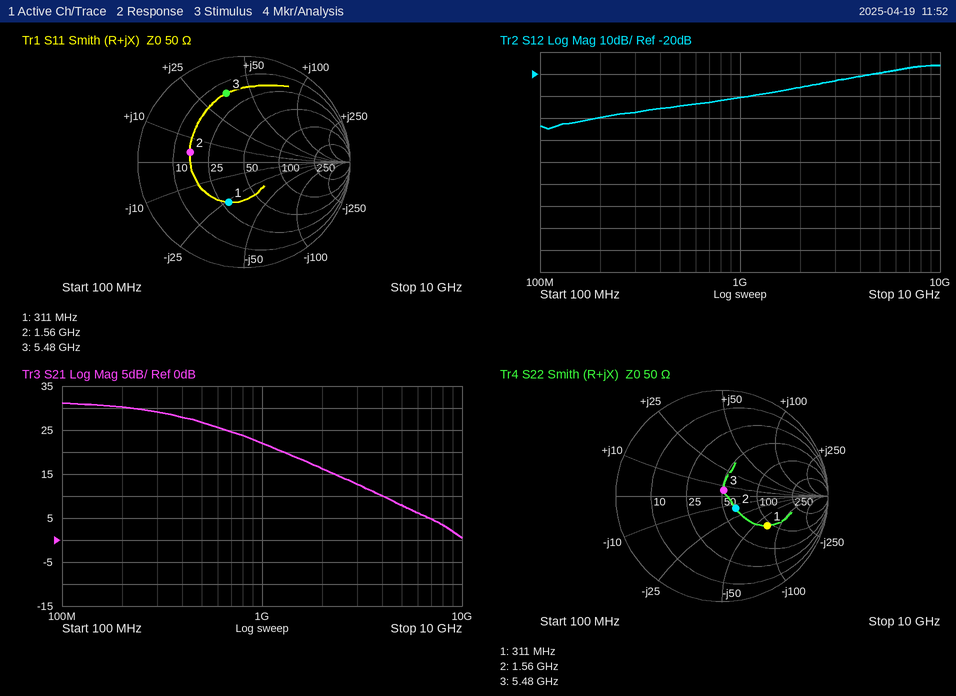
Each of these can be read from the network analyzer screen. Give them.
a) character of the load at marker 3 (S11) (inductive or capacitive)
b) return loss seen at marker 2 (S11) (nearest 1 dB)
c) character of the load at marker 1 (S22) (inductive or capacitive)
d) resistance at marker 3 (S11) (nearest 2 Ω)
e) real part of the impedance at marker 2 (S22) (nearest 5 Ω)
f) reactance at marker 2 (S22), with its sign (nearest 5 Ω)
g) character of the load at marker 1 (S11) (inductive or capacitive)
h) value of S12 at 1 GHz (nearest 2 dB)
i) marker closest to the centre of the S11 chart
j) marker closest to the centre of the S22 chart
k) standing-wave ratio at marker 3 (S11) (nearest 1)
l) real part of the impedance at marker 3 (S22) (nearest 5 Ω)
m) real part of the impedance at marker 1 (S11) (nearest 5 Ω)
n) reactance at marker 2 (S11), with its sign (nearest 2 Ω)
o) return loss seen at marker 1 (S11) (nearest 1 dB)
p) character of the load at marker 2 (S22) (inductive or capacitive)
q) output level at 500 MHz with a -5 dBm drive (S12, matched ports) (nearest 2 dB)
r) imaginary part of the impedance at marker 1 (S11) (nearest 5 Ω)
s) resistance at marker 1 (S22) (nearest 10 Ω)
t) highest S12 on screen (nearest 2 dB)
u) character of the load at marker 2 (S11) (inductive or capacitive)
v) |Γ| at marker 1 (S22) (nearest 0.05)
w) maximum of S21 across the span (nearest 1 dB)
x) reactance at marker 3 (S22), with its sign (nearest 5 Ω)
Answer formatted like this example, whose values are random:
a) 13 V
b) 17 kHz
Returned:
a) inductive
b) 6 dB
c) capacitive
d) 16 Ω
e) 65 Ω
f) -15 Ω
g) capacitive
h) -30 dB
i) marker 1
j) marker 3
k) 5
l) 50 Ω
m) 30 Ω
n) +4 Ω
o) 8 dB
p) capacitive
q) -40 dBm
r) -25 Ω
s) 90 Ω
t) -16 dB
u) inductive
v) 0.50
w) 31 dB
x) +5 Ω
